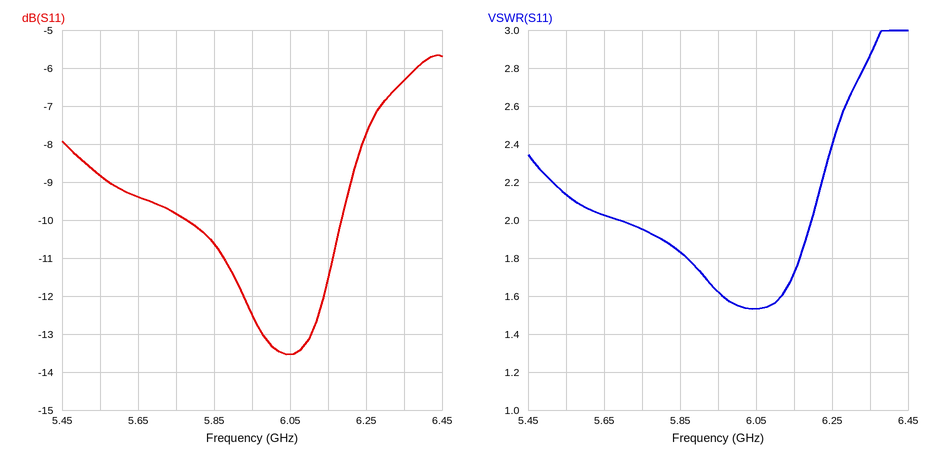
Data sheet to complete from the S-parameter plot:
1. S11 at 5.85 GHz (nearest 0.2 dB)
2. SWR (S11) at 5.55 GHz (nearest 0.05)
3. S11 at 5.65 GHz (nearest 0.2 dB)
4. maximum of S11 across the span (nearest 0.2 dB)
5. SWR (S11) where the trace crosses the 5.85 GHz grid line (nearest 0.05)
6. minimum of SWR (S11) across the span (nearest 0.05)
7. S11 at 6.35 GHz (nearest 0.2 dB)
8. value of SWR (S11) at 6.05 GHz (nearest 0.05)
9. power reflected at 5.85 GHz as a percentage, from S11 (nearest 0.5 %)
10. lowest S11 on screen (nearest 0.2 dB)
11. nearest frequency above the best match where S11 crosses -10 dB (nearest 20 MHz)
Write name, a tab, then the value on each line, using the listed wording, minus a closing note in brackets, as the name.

S11 at 5.85 GHz	-10.6 dB
SWR (S11) at 5.55 GHz	2.15
S11 at 5.65 GHz	-9.4 dB
maximum of S11 across the span	-5.6 dB
SWR (S11) where the trace crosses the 5.85 GHz grid line	1.85
minimum of SWR (S11) across the span	1.55
S11 at 6.35 GHz	-6.4 dB
value of SWR (S11) at 6.05 GHz	1.55
power reflected at 5.85 GHz as a percentage, from S11	8.5 %
lowest S11 on screen	-13.6 dB
nearest frequency above the best match where S11 crosses -10 dB	6.18 GHz
